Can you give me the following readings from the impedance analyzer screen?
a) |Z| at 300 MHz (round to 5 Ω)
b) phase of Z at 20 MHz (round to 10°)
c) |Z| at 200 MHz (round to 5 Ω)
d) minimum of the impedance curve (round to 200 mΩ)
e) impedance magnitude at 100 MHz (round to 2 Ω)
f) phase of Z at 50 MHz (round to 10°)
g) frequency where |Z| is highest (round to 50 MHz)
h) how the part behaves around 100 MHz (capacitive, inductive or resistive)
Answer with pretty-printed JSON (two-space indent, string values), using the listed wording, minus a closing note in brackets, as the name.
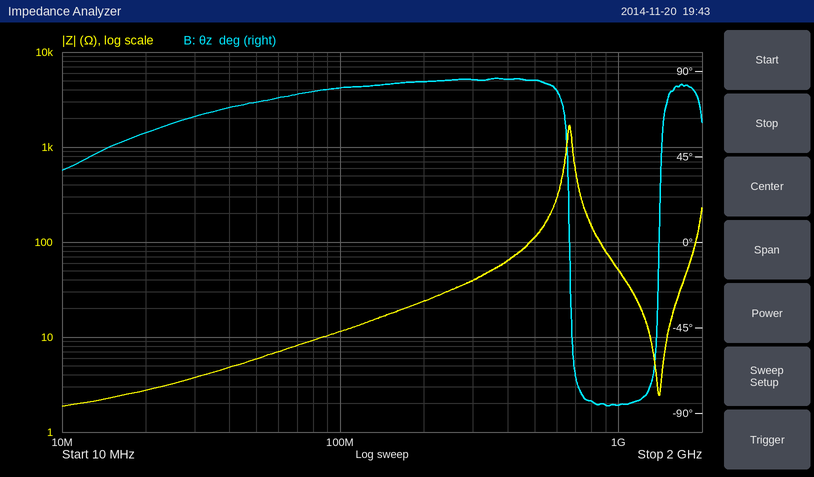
{
  "|Z| at 300 MHz": "40 Ω",
  "phase of Z at 20 MHz": "60°",
  "|Z| at 200 MHz": "25 Ω",
  "minimum of the impedance curve": "1.8 Ω",
  "impedance magnitude at 100 MHz": "12 Ω",
  "phase of Z at 50 MHz": "70°",
  "frequency where |Z| is highest": "650 MHz",
  "how the part behaves around 100 MHz": "inductive"
}
